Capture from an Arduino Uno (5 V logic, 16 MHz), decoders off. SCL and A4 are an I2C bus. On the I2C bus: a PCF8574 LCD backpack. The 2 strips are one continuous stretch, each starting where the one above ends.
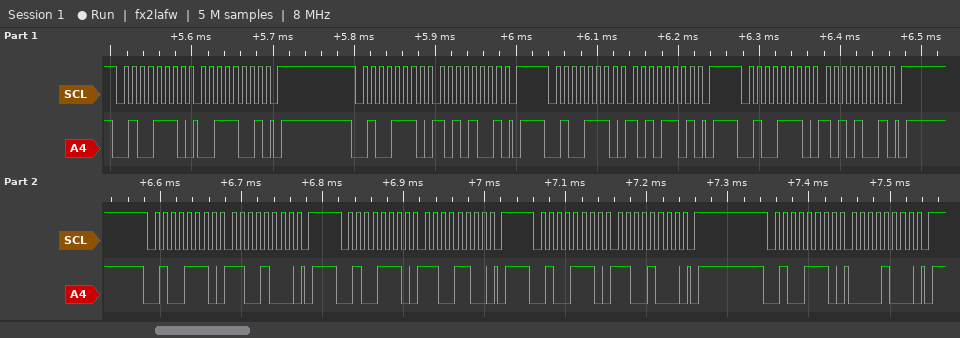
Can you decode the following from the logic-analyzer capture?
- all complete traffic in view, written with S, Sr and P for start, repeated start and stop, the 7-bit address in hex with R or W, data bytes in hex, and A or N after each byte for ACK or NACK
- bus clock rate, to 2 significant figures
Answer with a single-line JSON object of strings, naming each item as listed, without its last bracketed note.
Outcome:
{"all complete traffic in view, written with S, Sr and P for start, repeated start and stop, the 7-bit address in hex with R or W, data bytes in hex, and A or N after each byte for ACK or NACK": "S 27W A 39 A P S 27W A A9 A P S 27W A AD A P S 27W A A9 A P S 27W A C8 A P S 27W A CC A P S 27W A C8 A P S 27W A 08 A P", "bus clock rate, to 2 significant figures": "100 kHz"}
